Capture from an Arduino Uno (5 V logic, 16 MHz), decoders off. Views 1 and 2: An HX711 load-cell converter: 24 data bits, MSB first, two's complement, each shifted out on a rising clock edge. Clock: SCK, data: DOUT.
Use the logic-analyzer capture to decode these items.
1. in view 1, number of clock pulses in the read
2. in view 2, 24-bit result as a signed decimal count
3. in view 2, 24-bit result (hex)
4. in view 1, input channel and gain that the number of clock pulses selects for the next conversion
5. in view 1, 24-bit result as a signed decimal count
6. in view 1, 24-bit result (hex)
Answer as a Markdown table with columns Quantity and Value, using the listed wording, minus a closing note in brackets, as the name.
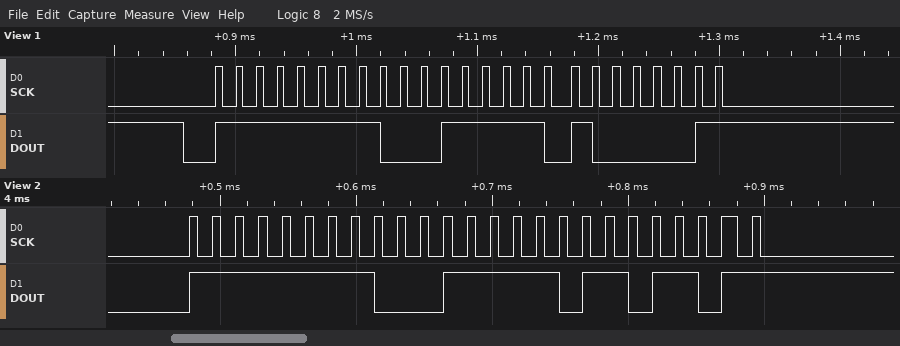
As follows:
| Quantity | Value |
|---|---|
| in view 1, number of clock pulses in the read | 25 |
| in view 2, 24-bit result as a signed decimal count | -57491 |
| in view 2, 24-bit result | 0xFF1F6D |
| in view 1, input channel and gain that the number of clock pulses selects for the next conversion | channel A, gain 128 |
| in view 1, 24-bit result as a signed decimal count | -57535 |
| in view 1, 24-bit result | 0xFF1F41 |
